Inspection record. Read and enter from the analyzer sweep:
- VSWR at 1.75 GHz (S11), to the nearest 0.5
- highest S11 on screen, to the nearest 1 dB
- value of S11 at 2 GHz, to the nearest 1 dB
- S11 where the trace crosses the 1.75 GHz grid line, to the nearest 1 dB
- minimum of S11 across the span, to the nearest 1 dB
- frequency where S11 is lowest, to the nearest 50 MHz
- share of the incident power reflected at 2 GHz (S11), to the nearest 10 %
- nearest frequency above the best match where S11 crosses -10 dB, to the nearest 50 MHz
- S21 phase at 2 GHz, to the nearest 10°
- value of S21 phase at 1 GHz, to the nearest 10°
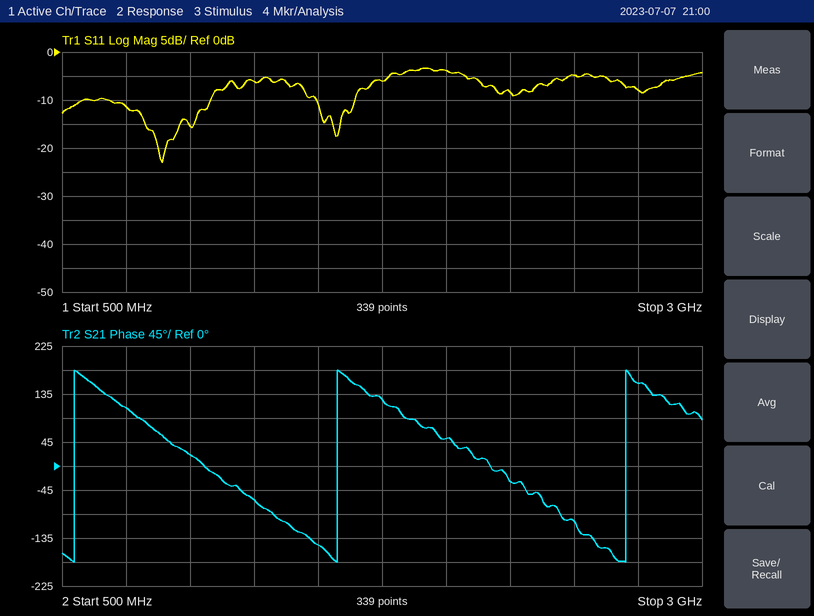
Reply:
3.0
-3 dB
-4 dB
-6 dB
-23 dB
900 MHz
40 %
1.10 GHz
50°
20°
